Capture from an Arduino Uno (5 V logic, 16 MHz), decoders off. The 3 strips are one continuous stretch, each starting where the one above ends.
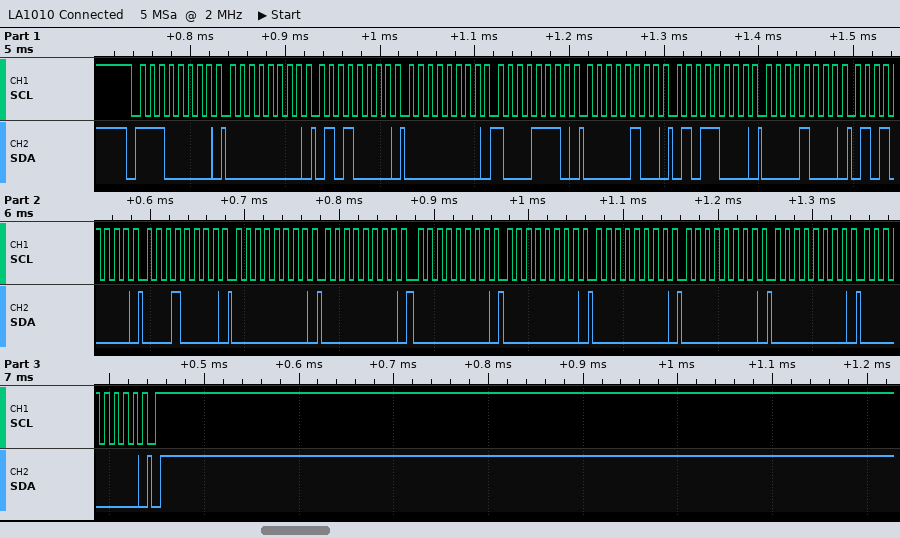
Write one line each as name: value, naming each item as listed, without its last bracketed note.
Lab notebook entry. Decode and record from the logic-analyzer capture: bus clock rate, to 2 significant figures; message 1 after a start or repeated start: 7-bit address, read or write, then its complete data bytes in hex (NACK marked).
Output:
bus clock rate, to 2 significant figures: 100 kHz
message 1 after a start or repeated start: 7-bit address, read or write, then its complete data bytes in hex: 0x70 write: 00 50 00 8E 04 58 08 50 10 00 00 00 00 00 00 00 00
